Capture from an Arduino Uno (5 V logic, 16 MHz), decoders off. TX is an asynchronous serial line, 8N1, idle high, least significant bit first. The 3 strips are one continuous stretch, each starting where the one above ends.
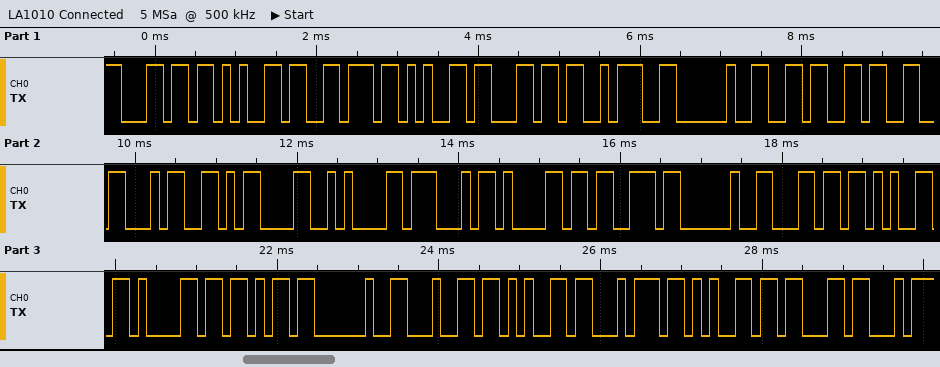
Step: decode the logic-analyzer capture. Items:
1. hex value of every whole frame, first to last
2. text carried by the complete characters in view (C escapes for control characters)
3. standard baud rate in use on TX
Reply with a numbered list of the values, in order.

1. 6C 65 76 65 6C 3A 20 36 33 34 0D 0A 47 61 73 20 6C 65 61 6B 20 64 65 74 65 63
2. "level: 634\r\nGas leak detec"
3. 9600 baud
